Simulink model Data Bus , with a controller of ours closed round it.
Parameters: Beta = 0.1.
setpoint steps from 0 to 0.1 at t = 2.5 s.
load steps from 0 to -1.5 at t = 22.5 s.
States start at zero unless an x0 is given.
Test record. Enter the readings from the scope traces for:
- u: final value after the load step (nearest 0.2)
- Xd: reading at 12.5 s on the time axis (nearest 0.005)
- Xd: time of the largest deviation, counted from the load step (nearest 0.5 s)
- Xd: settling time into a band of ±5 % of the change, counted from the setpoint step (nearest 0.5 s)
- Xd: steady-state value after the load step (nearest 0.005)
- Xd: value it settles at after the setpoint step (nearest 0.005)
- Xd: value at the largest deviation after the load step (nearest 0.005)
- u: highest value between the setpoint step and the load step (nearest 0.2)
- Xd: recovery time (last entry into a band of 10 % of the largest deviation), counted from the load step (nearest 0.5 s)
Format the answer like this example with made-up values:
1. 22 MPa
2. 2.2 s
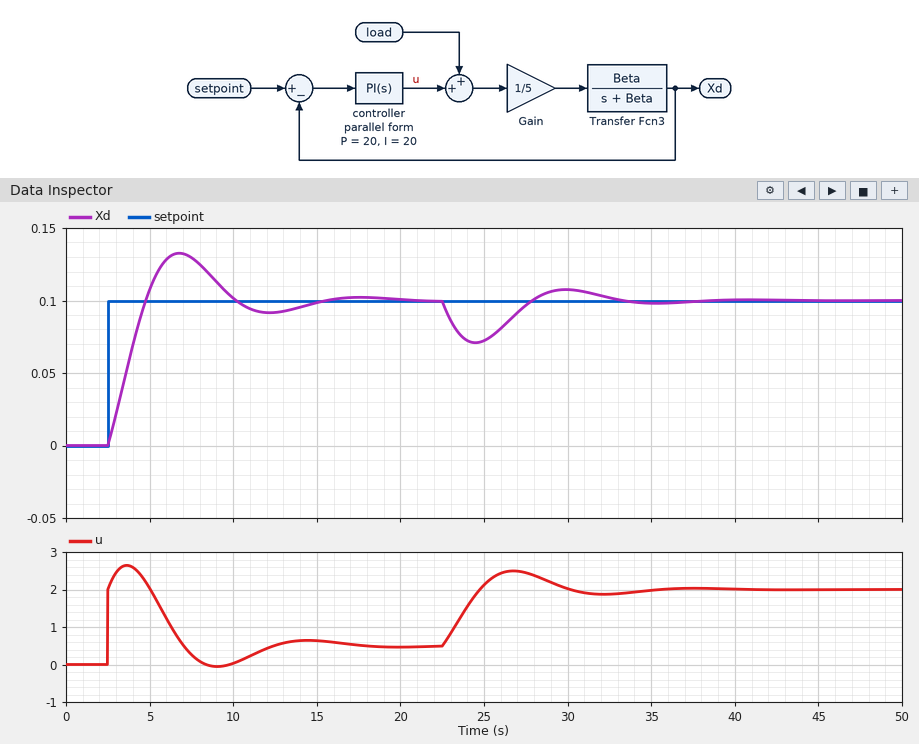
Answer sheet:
1. 2.0
2. 0.090
3. 2.0 s
4. 11.5 s
5. 0.100
6. 0.100
7. 0.070
8. 2.6
9. 9.5 s
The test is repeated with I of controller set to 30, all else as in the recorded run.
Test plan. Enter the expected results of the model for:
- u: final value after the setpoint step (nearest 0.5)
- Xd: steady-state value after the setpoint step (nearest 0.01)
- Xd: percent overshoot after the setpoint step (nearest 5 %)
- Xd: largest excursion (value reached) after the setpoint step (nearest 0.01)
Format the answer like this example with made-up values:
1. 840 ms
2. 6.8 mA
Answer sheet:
1. 0.5
2. 0.10
3. 40 %
4. 0.14
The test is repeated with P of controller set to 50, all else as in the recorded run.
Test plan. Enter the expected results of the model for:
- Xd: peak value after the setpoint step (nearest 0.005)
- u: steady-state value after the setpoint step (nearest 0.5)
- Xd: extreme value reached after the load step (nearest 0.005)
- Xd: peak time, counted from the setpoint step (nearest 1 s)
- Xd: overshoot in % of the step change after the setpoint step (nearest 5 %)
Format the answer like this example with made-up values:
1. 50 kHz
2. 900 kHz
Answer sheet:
1. 0.110
2. 0.5
3. 0.080
4. 4 s
5. 10 %
